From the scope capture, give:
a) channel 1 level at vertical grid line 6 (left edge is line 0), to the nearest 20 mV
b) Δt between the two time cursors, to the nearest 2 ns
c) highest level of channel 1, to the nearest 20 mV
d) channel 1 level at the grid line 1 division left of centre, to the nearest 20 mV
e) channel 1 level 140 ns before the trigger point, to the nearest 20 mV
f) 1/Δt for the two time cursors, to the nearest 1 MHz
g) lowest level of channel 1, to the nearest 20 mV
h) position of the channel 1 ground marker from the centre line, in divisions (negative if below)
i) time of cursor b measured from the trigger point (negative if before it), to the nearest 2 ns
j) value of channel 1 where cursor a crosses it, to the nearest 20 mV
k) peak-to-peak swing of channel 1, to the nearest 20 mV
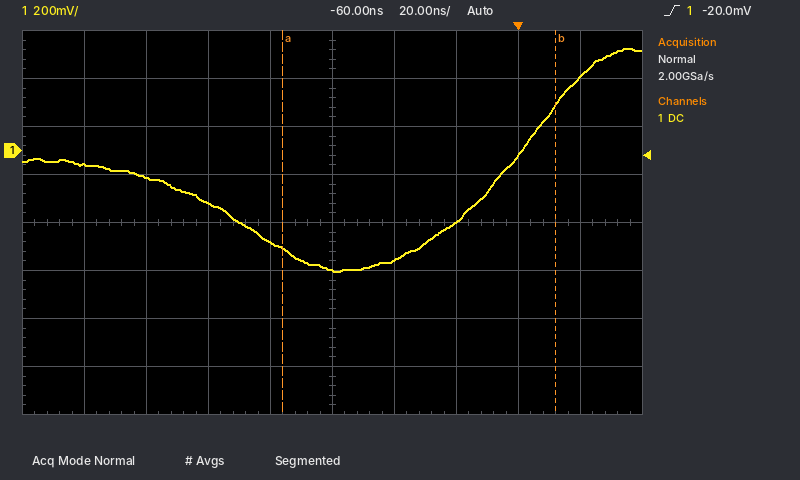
-460 mV
88 ns
420 mV
-380 mV
-60 mV
11 MHz
-500 mV
+1.5 div
+12 ns
-400 mV
920 mV
